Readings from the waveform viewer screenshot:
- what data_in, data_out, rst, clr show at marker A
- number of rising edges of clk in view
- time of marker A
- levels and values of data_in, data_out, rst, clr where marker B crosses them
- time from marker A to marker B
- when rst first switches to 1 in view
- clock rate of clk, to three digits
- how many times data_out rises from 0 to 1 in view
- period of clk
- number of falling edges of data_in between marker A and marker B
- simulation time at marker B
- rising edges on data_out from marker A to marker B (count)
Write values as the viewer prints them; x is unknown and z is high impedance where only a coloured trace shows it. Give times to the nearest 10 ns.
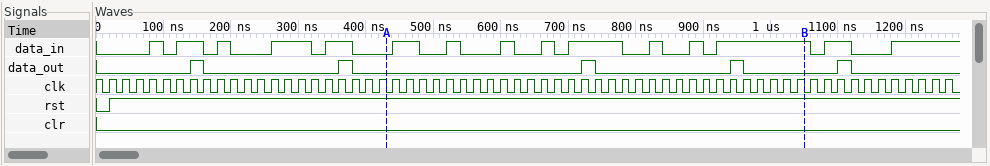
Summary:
data_in=0, data_out=0, rst=1, clr=0
63
430 ns
data_in=1, data_out=0, rst=1, clr=0
620 ns
20 ns
50.0 MHz
5
20 ns
7
1050 ns
2
